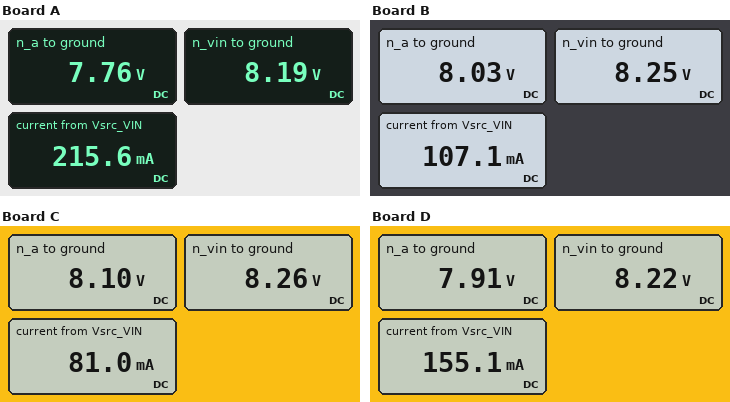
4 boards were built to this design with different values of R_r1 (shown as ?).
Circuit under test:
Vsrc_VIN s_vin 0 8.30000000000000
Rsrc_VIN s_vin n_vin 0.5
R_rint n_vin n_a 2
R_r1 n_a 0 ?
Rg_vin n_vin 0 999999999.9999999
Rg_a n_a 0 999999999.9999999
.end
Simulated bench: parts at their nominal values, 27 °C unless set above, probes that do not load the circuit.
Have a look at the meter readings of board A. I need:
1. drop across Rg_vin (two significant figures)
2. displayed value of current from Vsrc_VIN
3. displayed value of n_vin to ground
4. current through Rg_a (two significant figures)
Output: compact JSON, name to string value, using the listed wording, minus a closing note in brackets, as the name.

{"drop across Rg_vin": "8.2 V", "displayed value of current from Vsrc_VIN": "215.6 mA", "displayed value of n_vin to ground": "8.19 V", "current through Rg_a": "7.8 nA"}
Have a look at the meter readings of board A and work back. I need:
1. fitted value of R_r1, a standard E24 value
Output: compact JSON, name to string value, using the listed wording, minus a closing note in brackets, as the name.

{"fitted value of R_r1, a standard E24 value": "36 Ω"}
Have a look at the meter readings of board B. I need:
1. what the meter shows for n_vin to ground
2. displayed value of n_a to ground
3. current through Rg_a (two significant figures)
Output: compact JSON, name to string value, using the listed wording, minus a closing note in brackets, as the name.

{"what the meter shows for n_vin to ground": "8.25 V", "displayed value of n_a to ground": "8.03 V", "current through Rg_a": "8.0 nA"}
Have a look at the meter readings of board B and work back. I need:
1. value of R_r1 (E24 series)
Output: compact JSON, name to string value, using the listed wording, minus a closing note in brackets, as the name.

{"value of R_r1": "75 Ω"}
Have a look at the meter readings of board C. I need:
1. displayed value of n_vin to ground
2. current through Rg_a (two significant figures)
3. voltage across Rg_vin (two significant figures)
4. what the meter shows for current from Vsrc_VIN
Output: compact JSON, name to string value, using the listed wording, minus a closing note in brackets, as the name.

{"displayed value of n_vin to ground": "8.26 V", "current through Rg_a": "8.1 nA", "voltage across Rg_vin": "8.3 V", "what the meter shows for current from Vsrc_VIN": "81.0 mA"}
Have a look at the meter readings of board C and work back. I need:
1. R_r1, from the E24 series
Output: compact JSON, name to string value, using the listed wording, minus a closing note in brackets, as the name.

{"R_r1, from the E24 series": "100 Ω"}
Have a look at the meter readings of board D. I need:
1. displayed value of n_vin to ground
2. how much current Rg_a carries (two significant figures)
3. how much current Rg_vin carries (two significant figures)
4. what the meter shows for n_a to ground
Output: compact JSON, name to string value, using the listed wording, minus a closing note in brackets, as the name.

{"displayed value of n_vin to ground": "8.22 V", "how much current Rg_a carries": "7.9 nA", "how much current Rg_vin carries": "8.2 nA", "what the meter shows for n_a to ground": "7.91 V"}
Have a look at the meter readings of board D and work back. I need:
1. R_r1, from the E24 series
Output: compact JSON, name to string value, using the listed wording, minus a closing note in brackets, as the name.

{"R_r1, from the E24 series": "51 Ω"}
